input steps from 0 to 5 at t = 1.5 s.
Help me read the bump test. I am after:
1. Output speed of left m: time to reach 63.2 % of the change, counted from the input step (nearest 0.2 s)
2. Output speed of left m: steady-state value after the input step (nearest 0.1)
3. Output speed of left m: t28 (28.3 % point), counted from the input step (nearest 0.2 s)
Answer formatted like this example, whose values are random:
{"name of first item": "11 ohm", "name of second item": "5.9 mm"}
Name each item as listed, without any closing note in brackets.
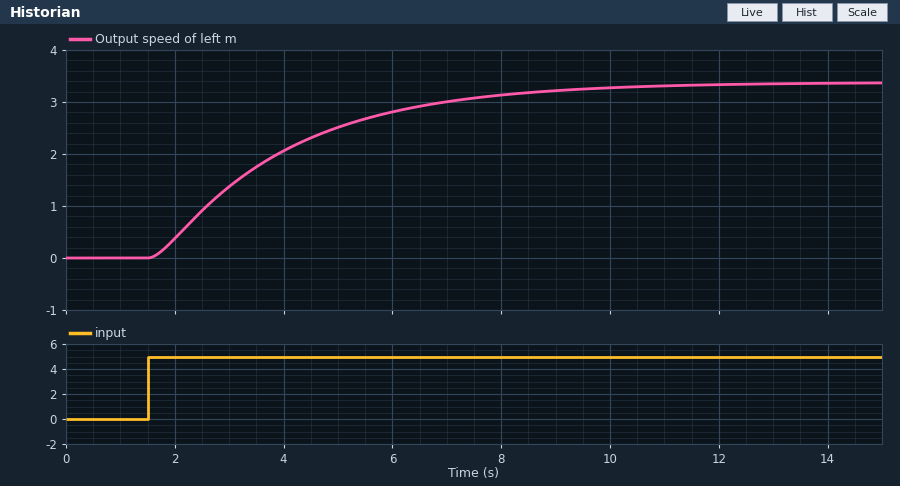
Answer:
{"Output speed of left m: time to reach 63.2 % of the change, counted from the input step": "2.6 s", "Output speed of left m: steady-state value after the input step": "3.4", "Output speed of left m: t28 (28.3 % point), counted from the input step": "1.0 s"}
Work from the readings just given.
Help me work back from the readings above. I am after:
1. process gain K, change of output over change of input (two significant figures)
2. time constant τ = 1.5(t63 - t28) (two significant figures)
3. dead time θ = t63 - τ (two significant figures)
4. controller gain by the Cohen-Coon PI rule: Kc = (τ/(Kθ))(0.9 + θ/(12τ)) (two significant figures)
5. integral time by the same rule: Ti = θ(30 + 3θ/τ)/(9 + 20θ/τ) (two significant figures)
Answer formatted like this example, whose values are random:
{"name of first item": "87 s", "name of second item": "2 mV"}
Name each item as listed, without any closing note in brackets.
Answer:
{"process gain K, change of output over change of input": "0.68", "time constant τ = 1.5(t63 - t28)": "2.4 s", "dead time θ = t63 - τ": "0.20 s", "controller gain by the Cohen-Coon PI rule: Kc = (τ/(Kθ))(0.9 + θ/(12τ))": "16", "integral time by the same rule: Ti = θ(30 + 3θ/τ)/(9 + 20θ/τ)": "0.57 s"}
